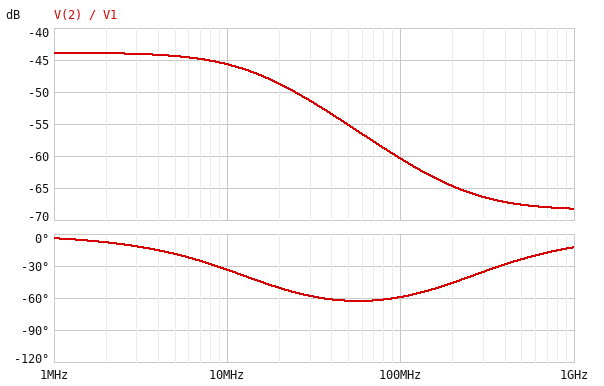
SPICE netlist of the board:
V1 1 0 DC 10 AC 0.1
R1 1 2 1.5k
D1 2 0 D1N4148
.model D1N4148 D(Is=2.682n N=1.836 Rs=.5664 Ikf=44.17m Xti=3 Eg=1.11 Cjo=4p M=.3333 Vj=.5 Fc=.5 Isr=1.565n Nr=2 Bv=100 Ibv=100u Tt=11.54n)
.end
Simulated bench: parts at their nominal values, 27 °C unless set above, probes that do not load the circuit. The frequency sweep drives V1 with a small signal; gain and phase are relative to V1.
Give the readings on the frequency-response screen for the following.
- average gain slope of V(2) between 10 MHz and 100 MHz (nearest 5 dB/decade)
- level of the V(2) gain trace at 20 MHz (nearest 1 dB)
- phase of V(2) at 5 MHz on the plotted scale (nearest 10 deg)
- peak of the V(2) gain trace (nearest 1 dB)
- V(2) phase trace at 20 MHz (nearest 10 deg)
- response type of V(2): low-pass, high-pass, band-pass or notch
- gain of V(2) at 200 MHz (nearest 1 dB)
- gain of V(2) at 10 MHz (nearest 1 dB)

-15 dB/decade
-49 dB
-20 deg
-44 dB
-50 deg
low-pass
-65 dB
-46 dB
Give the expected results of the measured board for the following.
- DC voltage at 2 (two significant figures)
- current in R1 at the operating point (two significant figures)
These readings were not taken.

710 mV
6.2 mA
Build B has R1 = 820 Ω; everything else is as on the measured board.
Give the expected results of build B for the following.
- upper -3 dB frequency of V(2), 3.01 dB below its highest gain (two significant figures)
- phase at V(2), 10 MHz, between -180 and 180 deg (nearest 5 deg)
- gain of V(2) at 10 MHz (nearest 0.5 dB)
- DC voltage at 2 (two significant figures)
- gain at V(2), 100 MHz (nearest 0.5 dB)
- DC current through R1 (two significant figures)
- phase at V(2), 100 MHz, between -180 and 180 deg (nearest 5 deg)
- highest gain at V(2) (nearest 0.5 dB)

14 MHz
-30 deg
-45.0 dB
750 mV
-58.5 dB
11 mA
-45 deg
-43.0 dB
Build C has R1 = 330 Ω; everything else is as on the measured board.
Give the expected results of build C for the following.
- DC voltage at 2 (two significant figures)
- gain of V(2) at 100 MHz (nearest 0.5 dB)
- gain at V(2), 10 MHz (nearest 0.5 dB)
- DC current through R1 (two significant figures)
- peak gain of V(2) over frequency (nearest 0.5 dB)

810 mV
-53.5 dB
-43.0 dB
28 mA
-41.0 dB
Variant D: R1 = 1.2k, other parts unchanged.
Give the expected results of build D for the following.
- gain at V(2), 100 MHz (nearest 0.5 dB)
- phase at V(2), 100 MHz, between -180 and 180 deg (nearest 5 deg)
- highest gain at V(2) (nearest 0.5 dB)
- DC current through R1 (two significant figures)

-60.0 dB
-55 deg
-43.5 dB
7.7 mA
